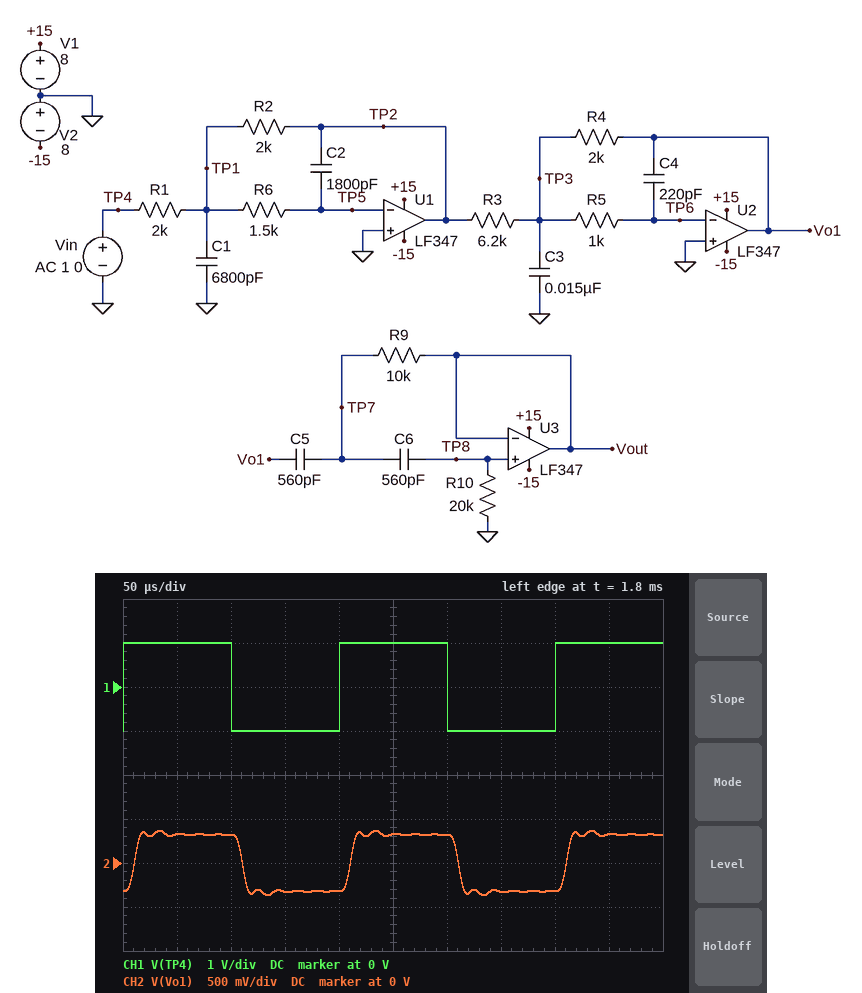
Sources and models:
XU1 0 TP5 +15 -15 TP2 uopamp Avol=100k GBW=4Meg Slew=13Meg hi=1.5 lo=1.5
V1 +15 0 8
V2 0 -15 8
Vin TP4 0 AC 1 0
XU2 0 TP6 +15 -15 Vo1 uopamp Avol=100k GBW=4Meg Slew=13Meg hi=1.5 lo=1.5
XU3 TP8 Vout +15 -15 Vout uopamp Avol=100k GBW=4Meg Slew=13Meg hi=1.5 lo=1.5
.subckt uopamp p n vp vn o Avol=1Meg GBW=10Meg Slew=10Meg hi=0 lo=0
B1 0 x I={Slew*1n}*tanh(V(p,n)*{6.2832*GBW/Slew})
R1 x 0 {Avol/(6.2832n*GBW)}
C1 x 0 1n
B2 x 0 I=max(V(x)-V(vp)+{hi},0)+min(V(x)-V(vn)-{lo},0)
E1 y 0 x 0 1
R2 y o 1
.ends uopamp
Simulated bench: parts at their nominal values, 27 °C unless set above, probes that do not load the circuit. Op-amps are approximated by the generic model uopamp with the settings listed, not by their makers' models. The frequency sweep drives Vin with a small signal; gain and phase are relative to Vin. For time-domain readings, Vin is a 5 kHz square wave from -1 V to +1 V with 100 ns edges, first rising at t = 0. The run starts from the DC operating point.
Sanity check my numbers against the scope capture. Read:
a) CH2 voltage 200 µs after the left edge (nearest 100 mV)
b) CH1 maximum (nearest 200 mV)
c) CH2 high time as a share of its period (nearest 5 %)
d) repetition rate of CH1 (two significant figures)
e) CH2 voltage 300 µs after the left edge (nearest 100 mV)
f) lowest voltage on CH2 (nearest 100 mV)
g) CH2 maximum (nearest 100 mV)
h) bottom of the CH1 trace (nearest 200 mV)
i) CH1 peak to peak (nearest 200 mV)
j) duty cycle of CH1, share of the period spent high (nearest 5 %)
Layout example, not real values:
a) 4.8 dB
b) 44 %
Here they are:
a) -300 mV
b) 1.0 V
c) 50 %
d) 5.0 kHz
e) 300 mV
f) -400 mV
g) 400 mV
h) -1.0 V
i) 2.0 V
j) 50 %
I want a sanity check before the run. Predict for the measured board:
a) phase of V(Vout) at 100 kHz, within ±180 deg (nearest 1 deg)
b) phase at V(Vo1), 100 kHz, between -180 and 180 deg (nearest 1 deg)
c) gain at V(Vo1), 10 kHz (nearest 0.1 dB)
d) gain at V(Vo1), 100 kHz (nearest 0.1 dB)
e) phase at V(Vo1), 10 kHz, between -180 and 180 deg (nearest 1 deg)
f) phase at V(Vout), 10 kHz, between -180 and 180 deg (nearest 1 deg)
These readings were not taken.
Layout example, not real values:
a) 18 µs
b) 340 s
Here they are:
a) 48 deg
b) 33 deg
c) -9.8 dB
d) -39.8 dB
e) -37 deg
f) 100 deg
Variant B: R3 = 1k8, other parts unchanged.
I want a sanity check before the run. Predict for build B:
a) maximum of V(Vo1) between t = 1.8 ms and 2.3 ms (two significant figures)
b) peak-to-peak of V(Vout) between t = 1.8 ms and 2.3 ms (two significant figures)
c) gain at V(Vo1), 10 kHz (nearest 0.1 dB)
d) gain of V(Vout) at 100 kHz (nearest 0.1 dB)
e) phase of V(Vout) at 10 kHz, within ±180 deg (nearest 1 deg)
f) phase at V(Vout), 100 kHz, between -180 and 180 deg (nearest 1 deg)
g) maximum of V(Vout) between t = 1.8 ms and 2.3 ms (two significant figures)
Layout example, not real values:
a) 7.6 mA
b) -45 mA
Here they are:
a) 1.2 V
b) 1.5 V
c) 1.0 dB
d) -29.3 dB
e) 99 deg
f) 51 deg
g) 770 mV
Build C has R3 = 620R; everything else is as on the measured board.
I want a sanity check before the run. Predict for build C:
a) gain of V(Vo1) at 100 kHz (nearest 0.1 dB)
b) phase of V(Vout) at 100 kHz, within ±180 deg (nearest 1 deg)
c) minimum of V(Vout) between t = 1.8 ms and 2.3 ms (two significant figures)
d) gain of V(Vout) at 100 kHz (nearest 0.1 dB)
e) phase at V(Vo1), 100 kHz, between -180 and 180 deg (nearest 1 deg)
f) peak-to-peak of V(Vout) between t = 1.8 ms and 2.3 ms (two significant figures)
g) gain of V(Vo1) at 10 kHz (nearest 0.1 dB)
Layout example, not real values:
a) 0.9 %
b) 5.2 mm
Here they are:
a) -20.4 dB
b) 59 deg
c) -2.0 V
d) -20.5 dB
e) 44 deg
f) 4.1 V
g) 10.2 dB
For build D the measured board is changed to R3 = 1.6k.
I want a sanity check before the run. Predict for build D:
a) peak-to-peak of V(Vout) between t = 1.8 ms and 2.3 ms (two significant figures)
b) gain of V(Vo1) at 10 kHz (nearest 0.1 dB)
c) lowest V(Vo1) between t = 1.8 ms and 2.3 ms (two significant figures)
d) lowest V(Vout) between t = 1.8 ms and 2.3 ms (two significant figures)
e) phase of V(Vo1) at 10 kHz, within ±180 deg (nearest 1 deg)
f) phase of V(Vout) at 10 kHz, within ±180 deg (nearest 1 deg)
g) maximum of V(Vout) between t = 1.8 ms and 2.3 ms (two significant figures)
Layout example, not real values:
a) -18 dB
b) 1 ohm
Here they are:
a) 1.7 V
b) 2.0 dB
c) -1.4 V
d) -860 mV
e) -38 deg
f) 99 deg
g) 860 mV
